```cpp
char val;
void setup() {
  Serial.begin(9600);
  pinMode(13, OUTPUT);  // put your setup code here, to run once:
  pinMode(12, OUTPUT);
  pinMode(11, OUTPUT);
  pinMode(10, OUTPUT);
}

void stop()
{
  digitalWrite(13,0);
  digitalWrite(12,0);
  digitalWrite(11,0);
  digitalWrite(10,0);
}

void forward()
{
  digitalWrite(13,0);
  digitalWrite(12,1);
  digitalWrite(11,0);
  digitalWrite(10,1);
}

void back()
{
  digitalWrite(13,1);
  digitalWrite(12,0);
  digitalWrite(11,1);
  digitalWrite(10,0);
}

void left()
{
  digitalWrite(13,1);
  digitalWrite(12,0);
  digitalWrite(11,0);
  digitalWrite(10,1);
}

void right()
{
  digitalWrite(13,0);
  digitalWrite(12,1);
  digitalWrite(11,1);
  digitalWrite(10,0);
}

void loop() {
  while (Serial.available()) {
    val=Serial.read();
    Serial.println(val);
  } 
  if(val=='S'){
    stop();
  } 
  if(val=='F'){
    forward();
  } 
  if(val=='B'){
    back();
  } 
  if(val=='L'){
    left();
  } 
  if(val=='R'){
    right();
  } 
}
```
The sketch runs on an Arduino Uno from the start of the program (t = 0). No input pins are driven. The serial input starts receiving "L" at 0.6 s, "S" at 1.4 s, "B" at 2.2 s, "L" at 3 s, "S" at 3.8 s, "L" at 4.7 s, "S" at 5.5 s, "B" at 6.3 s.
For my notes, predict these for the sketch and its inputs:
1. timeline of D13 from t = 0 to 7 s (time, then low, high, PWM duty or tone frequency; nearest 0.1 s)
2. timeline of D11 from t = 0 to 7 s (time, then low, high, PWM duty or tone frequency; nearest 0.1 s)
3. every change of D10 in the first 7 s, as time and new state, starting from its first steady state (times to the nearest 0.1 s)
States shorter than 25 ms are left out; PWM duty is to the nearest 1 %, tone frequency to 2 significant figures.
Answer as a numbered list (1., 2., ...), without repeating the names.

1. 0 s low; 0.6 s high; 1.4 s low; 2.2 s high; 3.8 s low; 4.7 s high; 5.5 s low; 6.3 s high
2. 0 s low; 2.2 s high; 3 s low; 6.3 s high
3. 0 s low; 0.6 s high; 1.4 s low; 3 s high; 3.8 s low; 4.7 s high; 5.5 s low
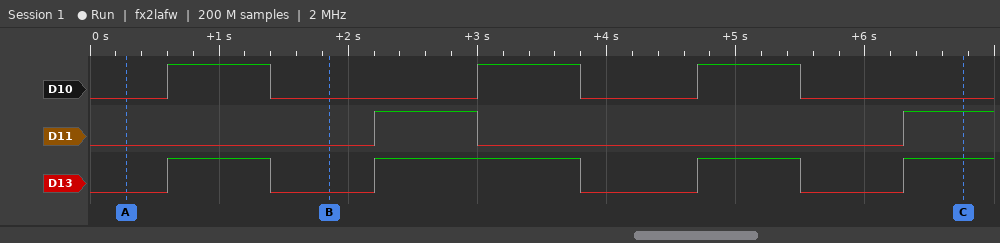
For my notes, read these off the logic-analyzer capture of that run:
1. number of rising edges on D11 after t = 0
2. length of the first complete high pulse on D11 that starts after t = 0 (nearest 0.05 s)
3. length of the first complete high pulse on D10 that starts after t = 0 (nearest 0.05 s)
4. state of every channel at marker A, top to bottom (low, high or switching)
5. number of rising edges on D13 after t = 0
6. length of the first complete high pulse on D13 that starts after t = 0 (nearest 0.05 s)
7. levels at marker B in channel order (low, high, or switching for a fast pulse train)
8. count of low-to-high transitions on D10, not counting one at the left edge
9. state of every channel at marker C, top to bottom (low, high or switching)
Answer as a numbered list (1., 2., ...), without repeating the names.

1. 2
2. 0.80 s
3. 0.80 s
4. D10 low, D11 low, D13 low
5. 4
6. 0.80 s
7. D10 low, D11 low, D13 low
8. 3
9. D10 low, D11 high, D13 high
